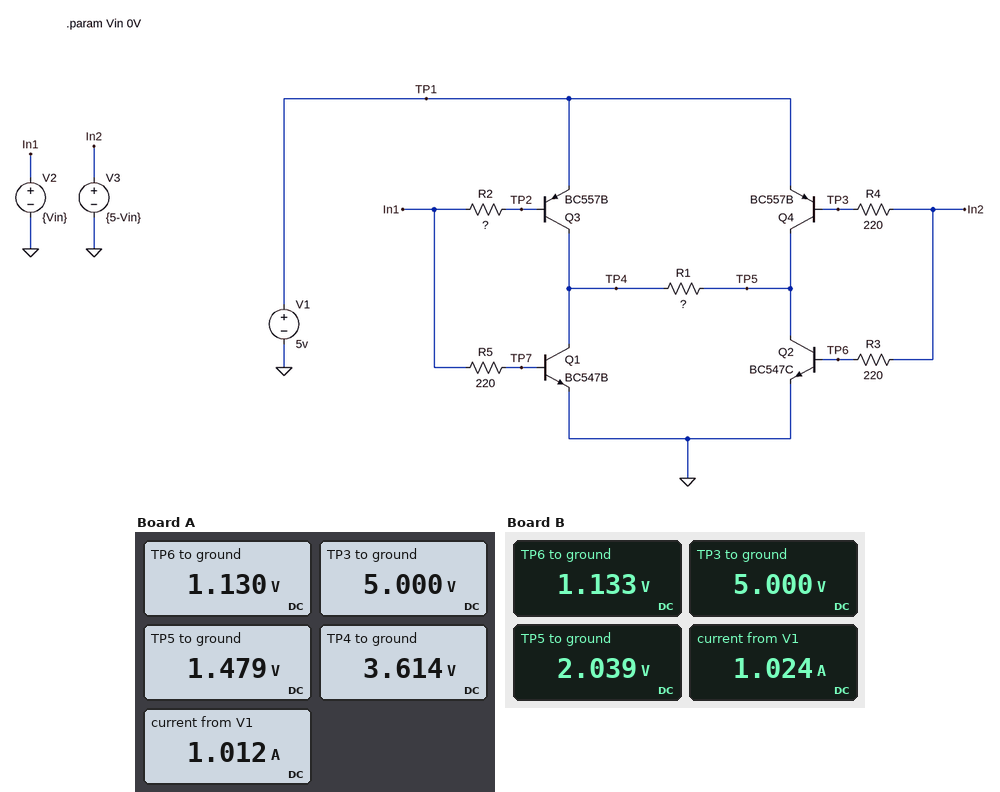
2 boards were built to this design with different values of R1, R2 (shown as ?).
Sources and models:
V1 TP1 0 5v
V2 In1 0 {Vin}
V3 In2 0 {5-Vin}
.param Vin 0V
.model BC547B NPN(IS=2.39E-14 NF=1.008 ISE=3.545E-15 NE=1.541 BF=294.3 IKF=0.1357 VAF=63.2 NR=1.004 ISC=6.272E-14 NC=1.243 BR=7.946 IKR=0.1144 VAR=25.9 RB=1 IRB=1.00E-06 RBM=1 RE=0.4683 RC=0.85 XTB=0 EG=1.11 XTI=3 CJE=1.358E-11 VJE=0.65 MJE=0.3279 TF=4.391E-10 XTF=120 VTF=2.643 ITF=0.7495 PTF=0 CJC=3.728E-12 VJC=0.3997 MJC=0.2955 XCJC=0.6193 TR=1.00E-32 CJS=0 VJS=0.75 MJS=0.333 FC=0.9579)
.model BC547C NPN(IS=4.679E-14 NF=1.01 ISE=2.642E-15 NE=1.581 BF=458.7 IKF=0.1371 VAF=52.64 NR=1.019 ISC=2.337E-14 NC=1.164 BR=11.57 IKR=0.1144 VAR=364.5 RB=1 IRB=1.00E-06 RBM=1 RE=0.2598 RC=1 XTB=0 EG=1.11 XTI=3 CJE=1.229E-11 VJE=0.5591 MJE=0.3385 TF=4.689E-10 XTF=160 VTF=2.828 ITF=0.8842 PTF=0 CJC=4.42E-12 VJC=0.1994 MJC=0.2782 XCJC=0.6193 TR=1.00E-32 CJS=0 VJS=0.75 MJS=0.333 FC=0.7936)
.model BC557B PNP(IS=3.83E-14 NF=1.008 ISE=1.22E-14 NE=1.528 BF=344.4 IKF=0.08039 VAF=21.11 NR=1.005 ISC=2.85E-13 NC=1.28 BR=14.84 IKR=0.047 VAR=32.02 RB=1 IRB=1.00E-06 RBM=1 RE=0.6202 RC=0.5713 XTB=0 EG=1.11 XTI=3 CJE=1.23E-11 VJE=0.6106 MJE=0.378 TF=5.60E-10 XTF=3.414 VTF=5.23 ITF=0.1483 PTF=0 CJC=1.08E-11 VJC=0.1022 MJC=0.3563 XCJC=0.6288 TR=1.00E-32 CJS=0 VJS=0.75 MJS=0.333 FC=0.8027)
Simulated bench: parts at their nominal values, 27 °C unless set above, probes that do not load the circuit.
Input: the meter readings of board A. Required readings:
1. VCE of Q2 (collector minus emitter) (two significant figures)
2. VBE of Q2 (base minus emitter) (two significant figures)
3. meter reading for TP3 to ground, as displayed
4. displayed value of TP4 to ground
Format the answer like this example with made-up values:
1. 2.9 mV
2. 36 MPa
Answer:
1. 1.5 V
2. 1.1 V
3. 5.000 V
4. 3.614 V
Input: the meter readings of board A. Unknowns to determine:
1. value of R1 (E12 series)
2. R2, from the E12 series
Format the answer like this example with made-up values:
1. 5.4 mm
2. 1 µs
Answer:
1. 2.2 Ω
2. 82 Ω
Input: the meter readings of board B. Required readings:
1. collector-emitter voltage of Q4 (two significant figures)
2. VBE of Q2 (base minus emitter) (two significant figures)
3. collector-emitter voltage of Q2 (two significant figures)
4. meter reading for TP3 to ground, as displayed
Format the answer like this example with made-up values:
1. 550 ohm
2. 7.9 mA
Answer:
1. -3.0 V
2. 1.1 V
3. 2.0 V
4. 5.000 V
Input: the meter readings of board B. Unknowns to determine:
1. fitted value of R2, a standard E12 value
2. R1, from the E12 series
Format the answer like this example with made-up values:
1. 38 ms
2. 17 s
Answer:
1. 82 Ω
2. 1.5 Ω
